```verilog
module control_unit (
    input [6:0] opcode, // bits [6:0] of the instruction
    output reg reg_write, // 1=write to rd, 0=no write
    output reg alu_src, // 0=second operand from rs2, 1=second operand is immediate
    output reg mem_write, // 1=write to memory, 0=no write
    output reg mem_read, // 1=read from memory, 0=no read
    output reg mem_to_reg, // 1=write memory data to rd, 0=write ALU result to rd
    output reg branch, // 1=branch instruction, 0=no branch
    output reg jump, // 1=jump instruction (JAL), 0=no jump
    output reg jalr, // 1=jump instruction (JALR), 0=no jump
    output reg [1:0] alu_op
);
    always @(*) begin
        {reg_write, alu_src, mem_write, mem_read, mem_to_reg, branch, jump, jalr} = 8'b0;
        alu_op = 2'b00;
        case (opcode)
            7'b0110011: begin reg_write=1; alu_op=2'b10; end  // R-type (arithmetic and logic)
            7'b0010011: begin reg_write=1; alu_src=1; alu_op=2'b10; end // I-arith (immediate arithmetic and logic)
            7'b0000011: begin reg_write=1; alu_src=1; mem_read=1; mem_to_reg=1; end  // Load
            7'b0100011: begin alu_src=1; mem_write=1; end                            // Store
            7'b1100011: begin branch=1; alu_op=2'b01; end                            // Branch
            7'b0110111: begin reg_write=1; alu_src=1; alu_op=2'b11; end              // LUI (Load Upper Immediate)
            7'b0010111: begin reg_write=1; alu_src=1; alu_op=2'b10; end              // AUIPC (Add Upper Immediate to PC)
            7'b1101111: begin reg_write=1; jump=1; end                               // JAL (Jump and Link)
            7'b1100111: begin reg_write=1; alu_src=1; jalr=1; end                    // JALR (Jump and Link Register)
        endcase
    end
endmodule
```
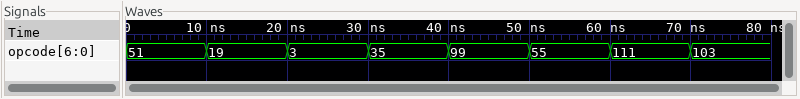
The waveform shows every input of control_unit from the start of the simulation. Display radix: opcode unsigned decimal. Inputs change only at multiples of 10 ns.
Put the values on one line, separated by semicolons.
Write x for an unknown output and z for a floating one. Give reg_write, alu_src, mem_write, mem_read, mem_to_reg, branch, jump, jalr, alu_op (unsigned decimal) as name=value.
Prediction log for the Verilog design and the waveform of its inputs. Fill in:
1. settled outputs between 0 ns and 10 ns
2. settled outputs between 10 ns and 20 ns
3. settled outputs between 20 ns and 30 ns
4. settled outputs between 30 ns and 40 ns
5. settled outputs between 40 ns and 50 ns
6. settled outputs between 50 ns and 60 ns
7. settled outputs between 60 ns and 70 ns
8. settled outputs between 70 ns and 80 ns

reg_write=1, alu_src=0, mem_write=0, mem_read=0, mem_to_reg=0, branch=0, jump=0, jalr=0, alu_op=2; reg_write=1, alu_src=1, mem_write=0, mem_read=0, mem_to_reg=0, branch=0, jump=0, jalr=0, alu_op=2; reg_write=1, alu_src=1, mem_write=0, mem_read=1, mem_to_reg=1, branch=0, jump=0, jalr=0, alu_op=0; reg_write=0, alu_src=1, mem_write=1, mem_read=0, mem_to_reg=0, branch=0, jump=0, jalr=0, alu_op=0; reg_write=0, alu_src=0, mem_write=0, mem_read=0, mem_to_reg=0, branch=1, jump=0, jalr=0, alu_op=1; reg_write=1, alu_src=1, mem_write=0, mem_read=0, mem_to_reg=0, branch=0, jump=0, jalr=0, alu_op=3; reg_write=1, alu_src=0, mem_write=0, mem_read=0, mem_to_reg=0, branch=0, jump=1, jalr=0, alu_op=0; reg_write=1, alu_src=1, mem_write=0, mem_read=0, mem_to_reg=0, branch=0, jump=0, jalr=1, alu_op=0
